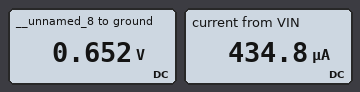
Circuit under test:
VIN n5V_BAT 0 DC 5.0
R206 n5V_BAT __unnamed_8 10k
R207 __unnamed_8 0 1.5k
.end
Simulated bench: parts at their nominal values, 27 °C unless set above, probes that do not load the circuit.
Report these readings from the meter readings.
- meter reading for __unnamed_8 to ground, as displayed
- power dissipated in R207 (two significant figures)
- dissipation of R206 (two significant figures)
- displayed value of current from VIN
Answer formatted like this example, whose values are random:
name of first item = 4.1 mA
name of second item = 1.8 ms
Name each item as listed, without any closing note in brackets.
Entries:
meter reading for __unnamed_8 to ground, as displayed = 0.652 V
power dissipated in R207 = 280 µW
dissipation of R206 = 1.9 mW
displayed value of current from VIN = 434.8 µA
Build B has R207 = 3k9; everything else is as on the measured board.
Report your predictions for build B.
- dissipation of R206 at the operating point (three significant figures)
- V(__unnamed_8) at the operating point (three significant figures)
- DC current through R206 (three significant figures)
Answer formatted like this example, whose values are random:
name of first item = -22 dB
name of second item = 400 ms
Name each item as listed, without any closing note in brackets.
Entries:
dissipation of R206 at the operating point = 1.29 mW
V(__unnamed_8) at the operating point = 1.40 V
DC current through R206 = 360 µA
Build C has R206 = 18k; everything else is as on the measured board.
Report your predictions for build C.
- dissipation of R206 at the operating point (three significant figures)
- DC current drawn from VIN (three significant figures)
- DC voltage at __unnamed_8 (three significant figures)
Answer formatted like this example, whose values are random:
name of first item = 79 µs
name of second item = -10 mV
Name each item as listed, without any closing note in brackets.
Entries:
dissipation of R206 at the operating point = 1.18 mW
DC current drawn from VIN = 256 µA
DC voltage at __unnamed_8 = 385 mV
